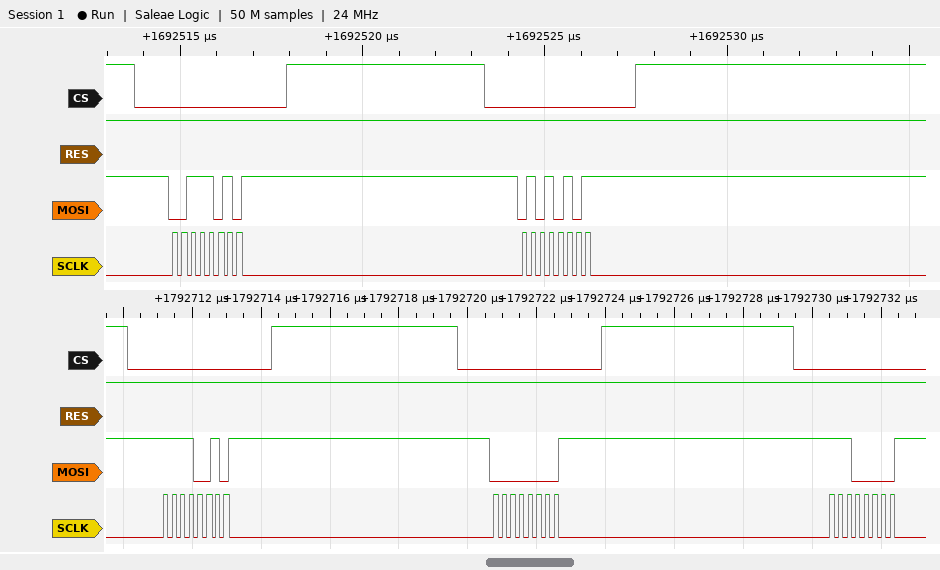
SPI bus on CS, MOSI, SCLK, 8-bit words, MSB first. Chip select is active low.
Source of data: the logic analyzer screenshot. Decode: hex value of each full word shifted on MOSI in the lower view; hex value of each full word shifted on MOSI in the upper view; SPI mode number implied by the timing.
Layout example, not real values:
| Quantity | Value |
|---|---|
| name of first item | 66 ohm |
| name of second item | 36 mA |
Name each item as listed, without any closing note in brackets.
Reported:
| Quantity | Value |
|---|---|
| hex value of each full word shifted on MOSI in the lower view | F2, 00, E0 |
| hex value of each full word shifted on MOSI in the upper view | 3A, 55 |
| SPI mode number implied by the timing | 0 |
